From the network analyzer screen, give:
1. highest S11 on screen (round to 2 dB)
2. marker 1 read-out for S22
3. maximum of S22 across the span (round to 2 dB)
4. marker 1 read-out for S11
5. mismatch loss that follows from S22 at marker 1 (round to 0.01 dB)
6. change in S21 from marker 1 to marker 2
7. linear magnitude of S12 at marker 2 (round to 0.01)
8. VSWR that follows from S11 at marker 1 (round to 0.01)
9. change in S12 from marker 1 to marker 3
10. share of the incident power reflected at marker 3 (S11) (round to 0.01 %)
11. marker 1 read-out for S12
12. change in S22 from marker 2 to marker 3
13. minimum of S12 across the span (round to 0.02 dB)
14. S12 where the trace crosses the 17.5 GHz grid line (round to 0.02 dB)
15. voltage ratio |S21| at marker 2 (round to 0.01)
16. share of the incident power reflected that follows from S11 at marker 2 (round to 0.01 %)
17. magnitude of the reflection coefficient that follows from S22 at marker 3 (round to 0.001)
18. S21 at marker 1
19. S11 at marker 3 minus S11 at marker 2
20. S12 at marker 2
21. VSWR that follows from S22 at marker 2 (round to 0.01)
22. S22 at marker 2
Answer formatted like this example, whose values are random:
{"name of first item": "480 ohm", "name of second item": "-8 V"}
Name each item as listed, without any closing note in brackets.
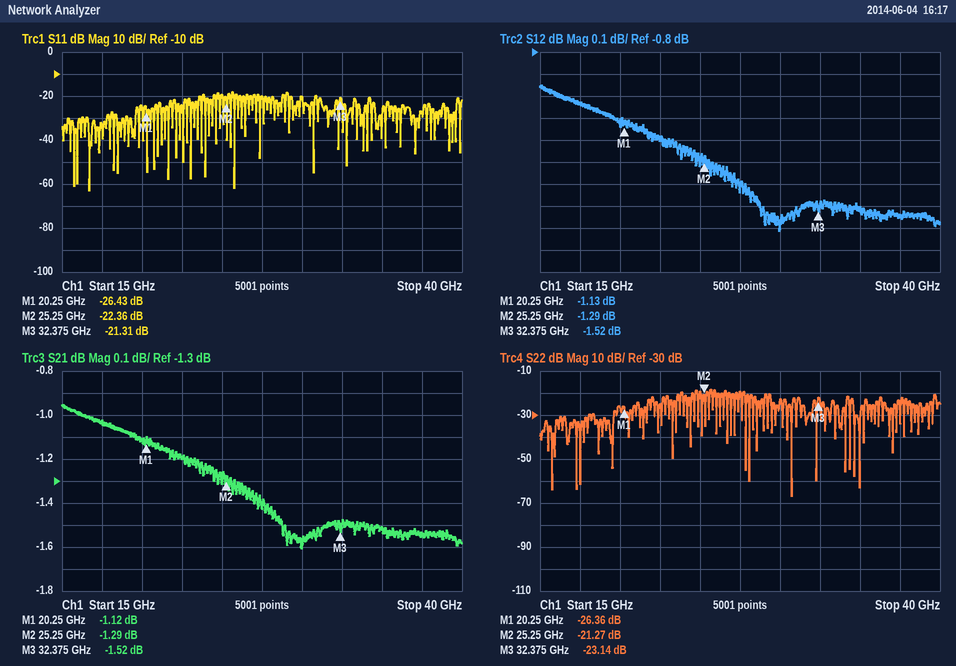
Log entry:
{"highest S11 on screen": "-18 dB", "marker 1 read-out for S22": "-26.36 dB", "maximum of S22 across the span": "-18 dB", "marker 1 read-out for S11": "-26.43 dB", "mismatch loss that follows from S22 at marker 1": "0.01 dB", "change in S21 from marker 1 to marker 2": "-0.17 dB", "linear magnitude of S12 at marker 2": "0.86", "VSWR that follows from S11 at marker 1": "1.10", "change in S12 from marker 1 to marker 3": "-0.39 dB", "share of the incident power reflected at marker 3 (S11)": "0.74 %", "marker 1 read-out for S12": "-1.13 dB", "change in S22 from marker 2 to marker 3": "-1.87 dB", "minimum of S12 across the span": "-1.62 dB", "S12 where the trace crosses the 17.5 GHz grid line": "-1.04 dB", "voltage ratio |S21| at marker 2": "0.86", "share of the incident power reflected that follows from S11 at marker 2": "0.58 %", "magnitude of the reflection coefficient that follows from S22 at marker 3": "0.070", "S21 at marker 1": "-1.12 dB", "S11 at marker 3 minus S11 at marker 2": "1.05 dB", "S12 at marker 2": "-1.29 dB", "VSWR that follows from S22 at marker 2": "1.19", "S22 at marker 2": "-21.27 dB"}
